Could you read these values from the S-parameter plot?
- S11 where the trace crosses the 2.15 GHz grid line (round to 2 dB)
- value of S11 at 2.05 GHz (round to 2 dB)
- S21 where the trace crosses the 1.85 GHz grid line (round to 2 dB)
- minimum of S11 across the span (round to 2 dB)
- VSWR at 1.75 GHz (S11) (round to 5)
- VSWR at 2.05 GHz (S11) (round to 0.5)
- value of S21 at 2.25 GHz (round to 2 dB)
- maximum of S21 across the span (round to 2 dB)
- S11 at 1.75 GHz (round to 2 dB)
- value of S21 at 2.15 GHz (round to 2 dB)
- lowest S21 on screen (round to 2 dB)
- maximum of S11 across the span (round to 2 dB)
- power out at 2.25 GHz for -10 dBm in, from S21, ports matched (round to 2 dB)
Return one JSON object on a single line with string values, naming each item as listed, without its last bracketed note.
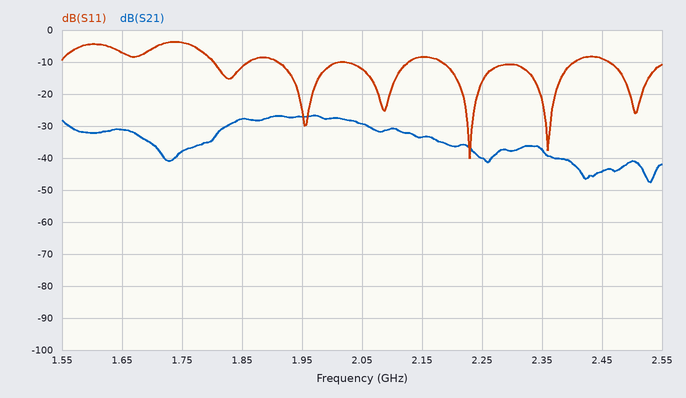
{"S11 where the trace crosses the 2.15 GHz grid line": "-8 dB", "value of S11 at 2.05 GHz": "-12 dB", "S21 where the trace crosses the 1.85 GHz grid line": "-28 dB", "minimum of S11 across the span": "-40 dB", "VSWR at 1.75 GHz (S11)": "5", "VSWR at 2.05 GHz (S11)": "1.5", "value of S21 at 2.25 GHz": "-40 dB", "maximum of S21 across the span": "-26 dB", "S11 at 1.75 GHz": "-4 dB", "value of S21 at 2.15 GHz": "-34 dB", "lowest S21 on screen": "-48 dB", "maximum of S11 across the span": "-4 dB", "power out at 2.25 GHz for -10 dBm in, from S21, ports matched": "-50 dBm"}
